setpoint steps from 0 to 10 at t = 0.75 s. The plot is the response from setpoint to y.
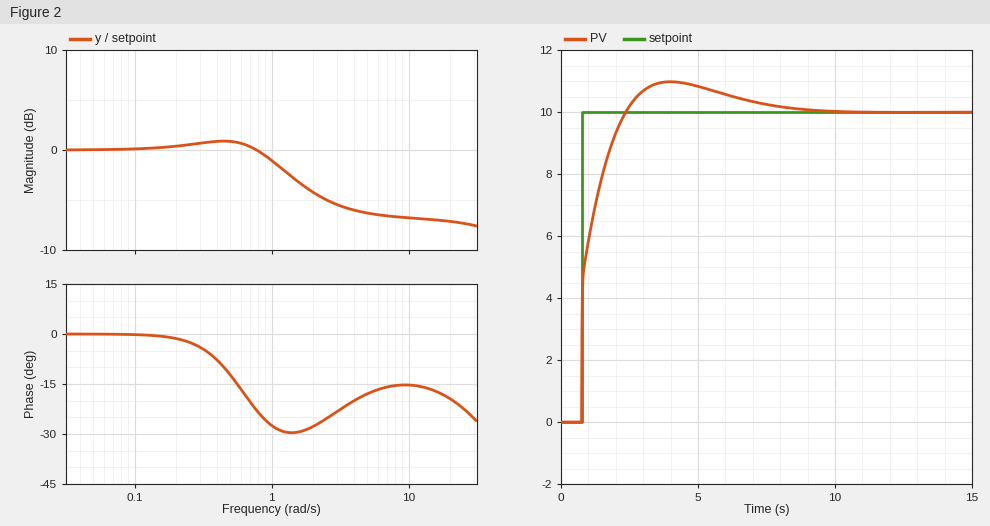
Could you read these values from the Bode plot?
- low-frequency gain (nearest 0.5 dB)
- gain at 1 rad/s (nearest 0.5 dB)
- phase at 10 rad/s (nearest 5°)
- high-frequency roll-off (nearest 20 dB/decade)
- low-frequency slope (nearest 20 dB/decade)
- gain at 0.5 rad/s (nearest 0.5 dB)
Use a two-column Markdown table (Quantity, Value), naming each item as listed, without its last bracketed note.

| Quantity | Value |
|---|---|
| low-frequency gain | 0.0 dB |
| gain at 1 rad/s | -1.0 dB |
| phase at 10 rad/s | -15° |
| high-frequency roll-off | 0 dB/decade |
| low-frequency slope | 0 dB/decade |
| gain at 0.5 rad/s | 1.0 dB |
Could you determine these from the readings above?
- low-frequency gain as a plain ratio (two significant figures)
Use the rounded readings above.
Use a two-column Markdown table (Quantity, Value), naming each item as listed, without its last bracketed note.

| Quantity | Value |
|---|---|
| low-frequency gain as a plain ratio | 1.0 |
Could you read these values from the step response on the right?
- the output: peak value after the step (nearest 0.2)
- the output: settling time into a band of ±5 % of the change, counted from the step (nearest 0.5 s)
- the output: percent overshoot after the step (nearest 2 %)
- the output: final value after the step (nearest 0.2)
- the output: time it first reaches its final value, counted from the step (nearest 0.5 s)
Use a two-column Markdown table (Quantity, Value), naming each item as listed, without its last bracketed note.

| Quantity | Value |
|---|---|
| the output: peak value after the step | 11.0 |
| the output: settling time into a band of ±5 % of the change, counted from the step | 5.5 s |
| the output: percent overshoot after the step | 10 % |
| the output: final value after the step | 10.0 |
| the output: time it first reaches its final value, counted from the step | 1.5 s |
